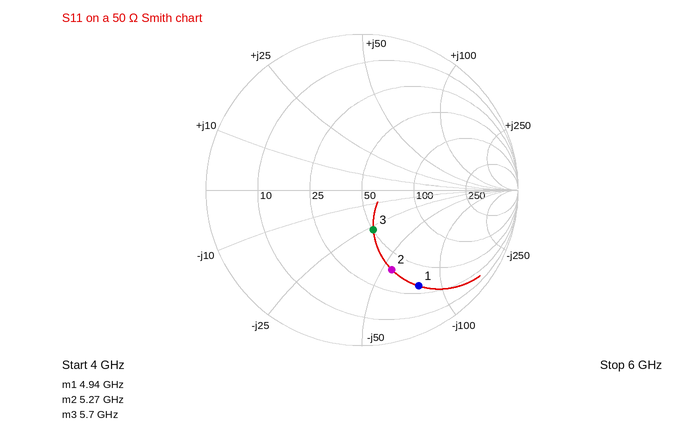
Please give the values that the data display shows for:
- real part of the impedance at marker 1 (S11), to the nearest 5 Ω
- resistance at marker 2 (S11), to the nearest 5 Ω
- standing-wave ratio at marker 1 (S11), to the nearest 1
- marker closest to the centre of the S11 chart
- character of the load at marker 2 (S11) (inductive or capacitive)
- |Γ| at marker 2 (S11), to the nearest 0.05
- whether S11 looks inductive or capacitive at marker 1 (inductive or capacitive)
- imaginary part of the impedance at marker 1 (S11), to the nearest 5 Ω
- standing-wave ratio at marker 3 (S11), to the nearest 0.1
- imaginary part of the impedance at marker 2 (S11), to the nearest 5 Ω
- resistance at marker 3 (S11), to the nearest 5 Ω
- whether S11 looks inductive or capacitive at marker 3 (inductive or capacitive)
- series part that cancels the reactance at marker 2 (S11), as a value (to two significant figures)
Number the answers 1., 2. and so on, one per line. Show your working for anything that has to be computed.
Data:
1. 30 Ω
2. 40 Ω
3. 6
4. marker 3
5. capacitive
6. 0.55
7. capacitive
8. -80 Ω
9. 1.7
10. -55 Ω
11. 50 Ω
12. capacitive
13. L = 55 Ω/(2π × 5.27 GHz) ≈ 1.7 nH
